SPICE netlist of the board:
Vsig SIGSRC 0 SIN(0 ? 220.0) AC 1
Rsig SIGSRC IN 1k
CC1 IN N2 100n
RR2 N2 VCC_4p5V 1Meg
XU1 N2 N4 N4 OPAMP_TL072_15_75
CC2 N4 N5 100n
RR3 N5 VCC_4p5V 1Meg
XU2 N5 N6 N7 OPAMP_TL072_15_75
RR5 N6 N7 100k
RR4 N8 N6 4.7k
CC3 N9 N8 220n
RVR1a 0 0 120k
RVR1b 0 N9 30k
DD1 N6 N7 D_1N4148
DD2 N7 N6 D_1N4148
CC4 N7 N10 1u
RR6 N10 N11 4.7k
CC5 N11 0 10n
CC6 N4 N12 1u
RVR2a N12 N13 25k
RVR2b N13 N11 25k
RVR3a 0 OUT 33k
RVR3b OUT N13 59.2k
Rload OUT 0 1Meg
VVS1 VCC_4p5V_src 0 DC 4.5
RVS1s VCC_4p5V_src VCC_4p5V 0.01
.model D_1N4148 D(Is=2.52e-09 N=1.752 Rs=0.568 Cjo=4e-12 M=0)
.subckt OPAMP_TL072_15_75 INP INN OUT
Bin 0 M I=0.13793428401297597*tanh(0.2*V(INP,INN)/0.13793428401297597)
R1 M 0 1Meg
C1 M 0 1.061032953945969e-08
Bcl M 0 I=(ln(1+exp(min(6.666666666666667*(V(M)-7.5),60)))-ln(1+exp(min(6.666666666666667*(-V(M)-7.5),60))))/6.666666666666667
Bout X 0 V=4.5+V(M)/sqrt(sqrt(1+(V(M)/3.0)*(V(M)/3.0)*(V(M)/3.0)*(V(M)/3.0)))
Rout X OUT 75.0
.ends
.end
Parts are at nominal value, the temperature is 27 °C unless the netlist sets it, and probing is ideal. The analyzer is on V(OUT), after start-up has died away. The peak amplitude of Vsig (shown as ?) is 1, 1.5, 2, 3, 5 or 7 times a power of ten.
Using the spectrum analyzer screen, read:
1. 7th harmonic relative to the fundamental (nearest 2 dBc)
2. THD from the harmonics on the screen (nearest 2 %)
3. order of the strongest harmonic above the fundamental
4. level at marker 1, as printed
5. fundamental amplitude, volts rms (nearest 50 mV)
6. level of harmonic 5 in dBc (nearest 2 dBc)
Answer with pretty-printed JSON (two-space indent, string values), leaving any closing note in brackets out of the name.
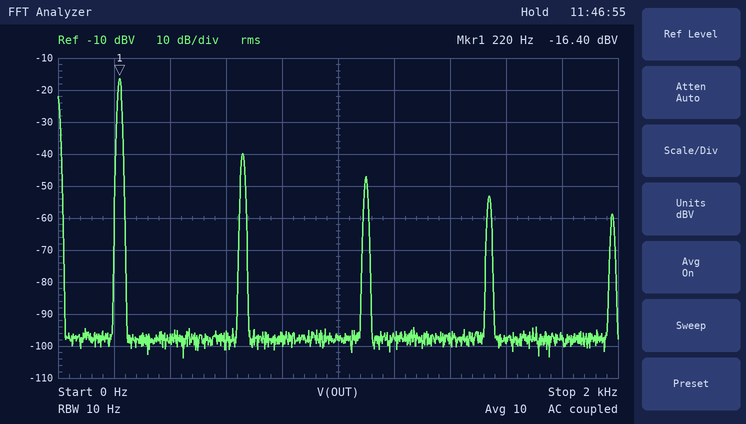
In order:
{
  "7th harmonic relative to the fundamental": "-36 dBc",
  "THD from the harmonics on the screen": "8 %",
  "order of the strongest harmonic above the fundamental": "3",
  "level at marker 1, as printed": "-16.40 dBV",
  "fundamental amplitude, volts rms": "150 mV",
  "level of harmonic 5 in dBc": "-30 dBc"
}
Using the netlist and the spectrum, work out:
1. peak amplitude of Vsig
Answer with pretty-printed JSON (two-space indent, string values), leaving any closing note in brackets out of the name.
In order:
{
  "peak amplitude of Vsig": "500 mV"
}
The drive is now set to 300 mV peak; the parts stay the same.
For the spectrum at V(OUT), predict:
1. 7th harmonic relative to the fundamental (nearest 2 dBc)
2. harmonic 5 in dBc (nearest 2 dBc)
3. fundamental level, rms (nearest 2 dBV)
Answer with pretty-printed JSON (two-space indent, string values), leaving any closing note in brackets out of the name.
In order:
{
  "7th harmonic relative to the fundamental": "-42 dBc",
  "harmonic 5 in dBc": "-32 dBc",
  "fundamental level, rms": "-20 dBV"
}
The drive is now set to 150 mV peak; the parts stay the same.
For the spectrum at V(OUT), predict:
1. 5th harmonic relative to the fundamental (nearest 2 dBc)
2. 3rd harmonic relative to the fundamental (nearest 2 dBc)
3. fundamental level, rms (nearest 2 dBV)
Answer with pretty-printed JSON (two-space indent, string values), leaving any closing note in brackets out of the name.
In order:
{
  "5th harmonic relative to the fundamental": "-46 dBc",
  "3rd harmonic relative to the fundamental": "-26 dBc",
  "fundamental level, rms": "-24 dBV"
}
